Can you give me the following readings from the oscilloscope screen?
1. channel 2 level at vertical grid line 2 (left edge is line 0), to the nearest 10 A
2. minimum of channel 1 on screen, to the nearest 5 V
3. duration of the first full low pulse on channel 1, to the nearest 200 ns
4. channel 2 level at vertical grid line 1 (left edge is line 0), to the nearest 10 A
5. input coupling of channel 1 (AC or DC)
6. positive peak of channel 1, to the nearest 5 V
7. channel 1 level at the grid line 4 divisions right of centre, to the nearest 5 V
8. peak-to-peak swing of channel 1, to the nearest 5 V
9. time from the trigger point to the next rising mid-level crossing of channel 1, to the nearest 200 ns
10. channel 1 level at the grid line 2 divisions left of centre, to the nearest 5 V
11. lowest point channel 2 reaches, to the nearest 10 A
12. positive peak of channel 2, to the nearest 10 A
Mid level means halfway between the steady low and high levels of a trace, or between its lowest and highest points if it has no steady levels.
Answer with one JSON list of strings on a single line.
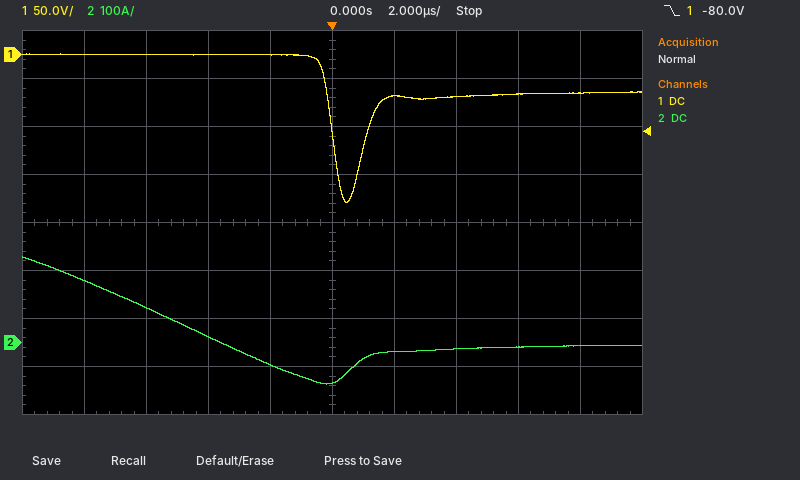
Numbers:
["70 A", "-155 V", "1.2 µs", "130 A", "DC", "0 V", "-40 V", "155 V", "1.2 µs", "0 V", "-90 A", "180 A"]
